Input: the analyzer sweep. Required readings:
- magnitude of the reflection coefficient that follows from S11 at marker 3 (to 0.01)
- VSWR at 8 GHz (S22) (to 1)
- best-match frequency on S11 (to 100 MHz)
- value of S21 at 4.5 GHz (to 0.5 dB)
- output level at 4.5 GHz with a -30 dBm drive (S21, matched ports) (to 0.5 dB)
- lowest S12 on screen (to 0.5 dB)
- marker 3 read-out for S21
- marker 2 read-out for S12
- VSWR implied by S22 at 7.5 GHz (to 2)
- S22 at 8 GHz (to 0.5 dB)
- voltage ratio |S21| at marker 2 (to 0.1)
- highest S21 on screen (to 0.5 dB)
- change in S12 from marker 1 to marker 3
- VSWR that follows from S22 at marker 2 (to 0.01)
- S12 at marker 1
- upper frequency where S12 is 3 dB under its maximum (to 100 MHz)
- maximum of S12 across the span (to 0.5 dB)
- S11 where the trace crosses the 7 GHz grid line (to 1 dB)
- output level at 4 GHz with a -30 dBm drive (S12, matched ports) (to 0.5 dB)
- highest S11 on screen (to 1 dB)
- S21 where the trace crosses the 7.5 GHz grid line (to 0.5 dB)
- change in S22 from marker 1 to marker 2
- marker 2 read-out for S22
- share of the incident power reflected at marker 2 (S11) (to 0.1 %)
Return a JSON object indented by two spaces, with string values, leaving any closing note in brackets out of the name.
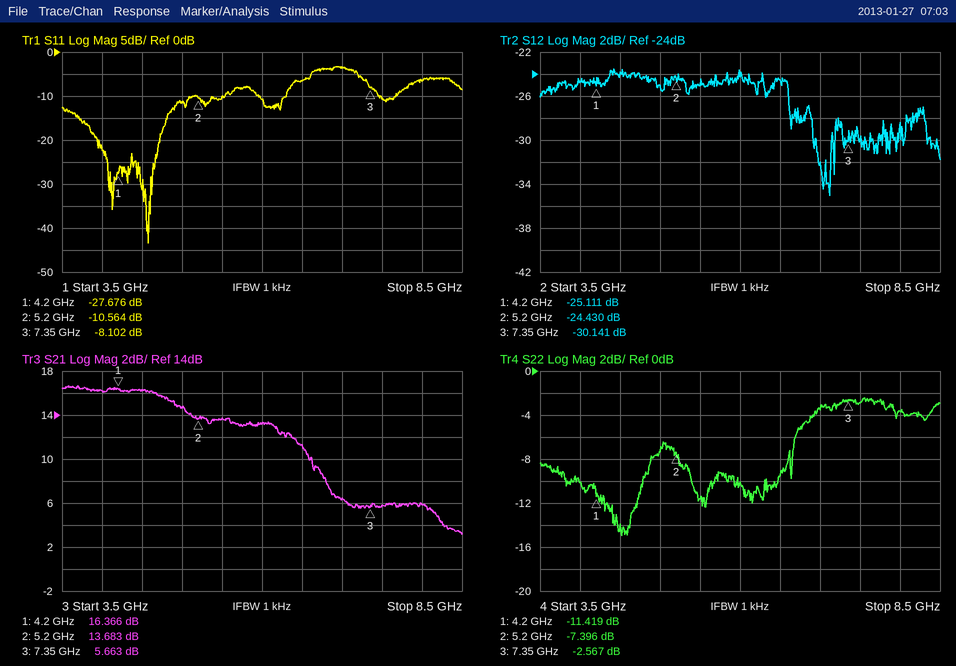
{
  "magnitude of the reflection coefficient that follows from S11 at marker 3": "0.39",
  "VSWR at 8 GHz (S22)": "5",
  "best-match frequency on S11": "4.6 GHz",
  "value of S21 at 4.5 GHz": "16.5 dB",
  "output level at 4.5 GHz with a -30 dBm drive (S21, matched ports)": "-13.5 dBm",
  "lowest S12 on screen": "-35.0 dB",
  "marker 3 read-out for S21": "5.663 dB",
  "marker 2 read-out for S12": "-24.430 dB",
  "VSWR implied by S22 at 7.5 GHz": "6",
  "S22 at 8 GHz": "-3.5 dB",
  "voltage ratio |S21| at marker 2": "4.8",
  "highest S21 on screen": "16.5 dB",
  "change in S12 from marker 1 to marker 3": "-5.030 dB",
  "VSWR that follows from S22 at marker 2": "2.49",
  "S12 at marker 1": "-25.111 dB",
  "upper frequency where S12 is 3 dB under its maximum": "6.6 GHz",
  "maximum of S12 across the span": "-23.5 dB",
  "S11 where the trace crosses the 7 GHz grid line": "-3 dB",
  "output level at 4 GHz with a -30 dBm drive (S12, matched ports)": "-54.5 dBm",
  "highest S11 on screen": "-3 dB",
  "S21 where the trace crosses the 7.5 GHz grid line": "6.0 dB",
  "change in S22 from marker 1 to marker 2": "4.023 dB",
  "marker 2 read-out for S22": "-7.396 dB",
  "share of the incident power reflected at marker 2 (S11)": "8.8 %"
}
